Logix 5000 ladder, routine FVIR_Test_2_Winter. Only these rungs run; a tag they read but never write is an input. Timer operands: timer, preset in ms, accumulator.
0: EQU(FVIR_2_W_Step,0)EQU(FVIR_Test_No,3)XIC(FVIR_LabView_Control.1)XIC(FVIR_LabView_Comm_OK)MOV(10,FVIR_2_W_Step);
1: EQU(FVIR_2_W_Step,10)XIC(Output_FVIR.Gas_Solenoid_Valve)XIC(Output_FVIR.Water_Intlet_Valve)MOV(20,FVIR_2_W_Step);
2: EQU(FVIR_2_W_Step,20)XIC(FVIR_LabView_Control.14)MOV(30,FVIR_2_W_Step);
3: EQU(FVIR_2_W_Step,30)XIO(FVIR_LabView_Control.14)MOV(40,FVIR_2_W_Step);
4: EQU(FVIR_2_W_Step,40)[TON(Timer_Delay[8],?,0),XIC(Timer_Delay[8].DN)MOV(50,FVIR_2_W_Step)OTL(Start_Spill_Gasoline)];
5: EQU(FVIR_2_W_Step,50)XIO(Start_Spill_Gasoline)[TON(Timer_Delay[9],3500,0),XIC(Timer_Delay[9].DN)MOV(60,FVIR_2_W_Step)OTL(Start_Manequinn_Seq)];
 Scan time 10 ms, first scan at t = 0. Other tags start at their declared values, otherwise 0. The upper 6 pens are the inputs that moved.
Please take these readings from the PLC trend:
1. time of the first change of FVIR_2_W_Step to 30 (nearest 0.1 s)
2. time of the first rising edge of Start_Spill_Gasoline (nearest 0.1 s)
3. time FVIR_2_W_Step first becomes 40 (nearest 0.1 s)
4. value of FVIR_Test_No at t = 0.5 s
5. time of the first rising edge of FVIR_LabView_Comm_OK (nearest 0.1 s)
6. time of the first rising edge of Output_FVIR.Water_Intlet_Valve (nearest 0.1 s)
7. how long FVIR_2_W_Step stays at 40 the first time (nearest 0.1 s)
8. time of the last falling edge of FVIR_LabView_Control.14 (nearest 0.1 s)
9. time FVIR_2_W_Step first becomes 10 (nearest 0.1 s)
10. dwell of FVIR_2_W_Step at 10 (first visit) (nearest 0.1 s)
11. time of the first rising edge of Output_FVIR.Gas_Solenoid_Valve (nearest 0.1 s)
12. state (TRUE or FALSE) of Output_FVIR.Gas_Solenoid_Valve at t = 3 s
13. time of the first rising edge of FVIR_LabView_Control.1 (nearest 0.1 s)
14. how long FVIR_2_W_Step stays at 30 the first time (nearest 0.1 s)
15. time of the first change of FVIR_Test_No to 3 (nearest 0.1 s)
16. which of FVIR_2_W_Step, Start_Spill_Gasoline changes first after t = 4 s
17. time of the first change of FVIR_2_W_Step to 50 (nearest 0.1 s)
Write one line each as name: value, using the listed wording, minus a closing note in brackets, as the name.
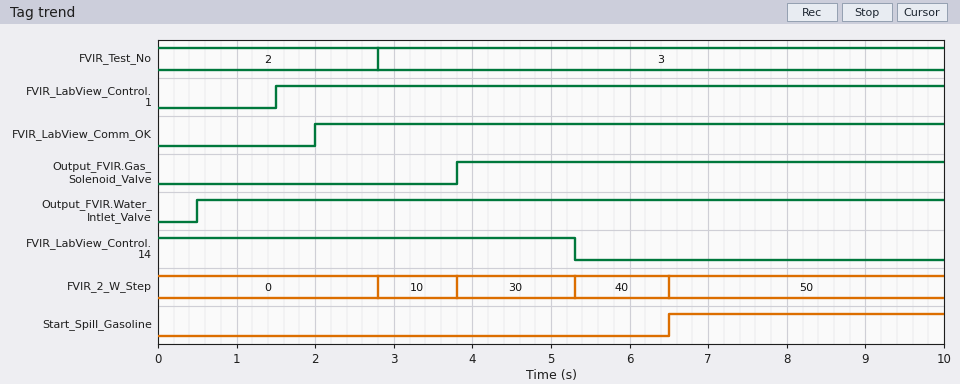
time of the first change of FVIR_2_W_Step to 30: 3.8 s
time of the first rising edge of Start_Spill_Gasoline: 6.5 s
time FVIR_2_W_Step first becomes 40: 5.3 s
value of FVIR_Test_No at t = 0.5 s: 2
time of the first rising edge of FVIR_LabView_Comm_OK: 2.0 s
time of the first rising edge of Output_FVIR.Water_Intlet_Valve: 0.5 s
how long FVIR_2_W_Step stays at 40 the first time: 1.2 s
time of the last falling edge of FVIR_LabView_Control.14: 5.3 s
time FVIR_2_W_Step first becomes 10: 2.8 s
dwell of FVIR_2_W_Step at 10 (first visit): 1.0 s
time of the first rising edge of Output_FVIR.Gas_Solenoid_Valve: 3.8 s
state (TRUE or FALSE) of Output_FVIR.Gas_Solenoid_Valve at t = 3 s: FALSE
time of the first rising edge of FVIR_LabView_Control.1: 1.5 s
how long FVIR_2_W_Step stays at 30 the first time: 1.5 s
time of the first change of FVIR_Test_No to 3: 2.8 s
which of FVIR_2_W_Step, Start_Spill_Gasoline changes first after t = 4 s: FVIR_2_W_Step
time of the first change of FVIR_2_W_Step to 50: 6.5 s
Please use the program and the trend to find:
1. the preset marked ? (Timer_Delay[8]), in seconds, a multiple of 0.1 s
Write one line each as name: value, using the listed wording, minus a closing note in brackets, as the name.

the preset marked ? (Timer_Delay[8]), in seconds, a multiple of 0.1 s: 1.2 s
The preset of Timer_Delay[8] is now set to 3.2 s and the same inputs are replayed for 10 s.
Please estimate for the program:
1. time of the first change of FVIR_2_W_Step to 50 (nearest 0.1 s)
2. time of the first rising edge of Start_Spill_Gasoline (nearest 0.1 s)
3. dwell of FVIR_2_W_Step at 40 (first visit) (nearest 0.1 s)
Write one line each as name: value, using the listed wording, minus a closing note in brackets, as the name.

time of the first change of FVIR_2_W_Step to 50: 8.5 s
time of the first rising edge of Start_Spill_Gasoline: 8.5 s
dwell of FVIR_2_W_Step at 40 (first visit): 3.2 s
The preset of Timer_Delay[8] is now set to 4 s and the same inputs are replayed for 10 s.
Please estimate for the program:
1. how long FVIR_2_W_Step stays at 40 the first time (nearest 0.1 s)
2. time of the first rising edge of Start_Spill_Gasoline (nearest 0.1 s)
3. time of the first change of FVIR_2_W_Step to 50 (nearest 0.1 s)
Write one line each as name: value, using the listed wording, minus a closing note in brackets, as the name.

how long FVIR_2_W_Step stays at 40 the first time: 4.0 s
time of the first rising edge of Start_Spill_Gasoline: 9.3 s
time of the first change of FVIR_2_W_Step to 50: 9.3 s
